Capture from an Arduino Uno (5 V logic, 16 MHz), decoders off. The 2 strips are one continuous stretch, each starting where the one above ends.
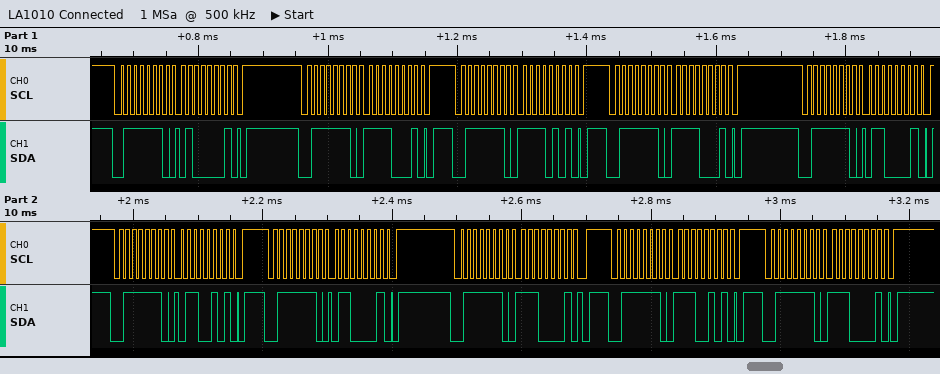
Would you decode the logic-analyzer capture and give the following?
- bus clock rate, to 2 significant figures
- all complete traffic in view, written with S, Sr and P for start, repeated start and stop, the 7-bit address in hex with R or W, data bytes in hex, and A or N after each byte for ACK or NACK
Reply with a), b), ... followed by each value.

a) 100 kHz
b) S 3FW A 41 A P S 3FW A F1 A P S 3FW A F5 A P S 3FW A F1 A P S 3FW A 61 A P S 3FW A 65 A P S 3FW A 61 A P S 3FW A E1 A P S 3FW A E5 A P S 3FW A E1 A P
